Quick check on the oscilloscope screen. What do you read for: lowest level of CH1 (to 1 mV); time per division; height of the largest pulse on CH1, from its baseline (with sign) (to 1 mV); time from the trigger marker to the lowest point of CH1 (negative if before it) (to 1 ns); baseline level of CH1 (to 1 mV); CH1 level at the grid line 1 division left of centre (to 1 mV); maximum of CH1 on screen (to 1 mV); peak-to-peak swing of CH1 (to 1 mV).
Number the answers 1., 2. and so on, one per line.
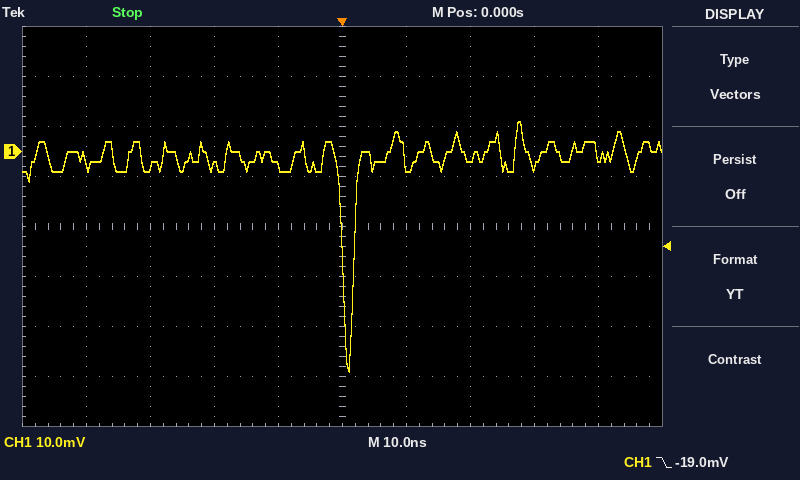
1. -44 mV
2. 10 ns
3. -43 mV
4. +1 ns
5. -1 mV
6. -3 mV
7. 6 mV
8. 50 mV
